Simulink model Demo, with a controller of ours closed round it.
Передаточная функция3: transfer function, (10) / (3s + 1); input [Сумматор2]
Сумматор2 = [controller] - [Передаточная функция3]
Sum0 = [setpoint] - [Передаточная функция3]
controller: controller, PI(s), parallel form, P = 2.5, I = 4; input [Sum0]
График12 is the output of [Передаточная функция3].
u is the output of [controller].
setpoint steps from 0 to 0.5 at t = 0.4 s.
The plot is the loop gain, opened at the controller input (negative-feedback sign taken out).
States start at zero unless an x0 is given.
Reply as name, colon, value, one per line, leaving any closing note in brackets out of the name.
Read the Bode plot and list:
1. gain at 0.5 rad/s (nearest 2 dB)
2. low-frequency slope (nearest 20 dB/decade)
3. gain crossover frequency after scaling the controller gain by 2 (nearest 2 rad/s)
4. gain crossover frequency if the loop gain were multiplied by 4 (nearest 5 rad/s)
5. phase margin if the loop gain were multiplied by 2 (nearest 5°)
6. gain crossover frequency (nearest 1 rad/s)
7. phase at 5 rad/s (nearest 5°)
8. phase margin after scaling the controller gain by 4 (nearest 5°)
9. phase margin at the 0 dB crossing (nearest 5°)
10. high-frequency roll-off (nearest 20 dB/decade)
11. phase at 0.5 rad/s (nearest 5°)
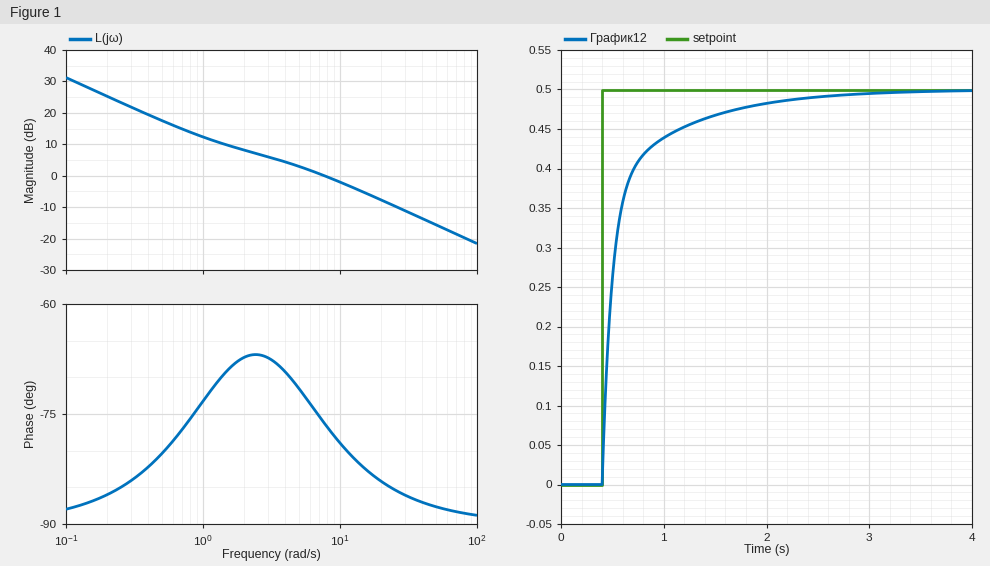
gain at 0.5 rad/s: 18 dB
low-frequency slope: -20 dB/decade
gain crossover frequency after scaling the controller gain by 2: 16 rad/s
gain crossover frequency if the loop gain were multiplied by 4: 35 rad/s
phase margin if the loop gain were multiplied by 2: 95°
gain crossover frequency: 8 rad/s
phase at 5 rad/s: -70°
phase margin after scaling the controller gain by 4: 95°
phase margin at the 0 dB crossing: 105°
high-frequency roll-off: -20 dB/decade
phase at 0.5 rad/s: -80°
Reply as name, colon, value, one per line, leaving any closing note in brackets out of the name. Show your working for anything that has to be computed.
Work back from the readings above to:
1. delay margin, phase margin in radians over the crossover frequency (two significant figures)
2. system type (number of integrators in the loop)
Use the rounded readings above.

delay margin, phase margin in radians over the crossover frequency: 105 × π / 180 / 8 = 0.23 s
system type: 1
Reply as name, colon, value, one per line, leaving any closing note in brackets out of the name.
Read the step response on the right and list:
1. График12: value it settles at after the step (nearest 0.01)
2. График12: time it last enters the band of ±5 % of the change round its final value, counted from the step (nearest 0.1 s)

График12: value it settles at after the step: 0.50
График12: time it last enters the band of ±5 % of the change round its final value, counted from the step: 1.3 s
